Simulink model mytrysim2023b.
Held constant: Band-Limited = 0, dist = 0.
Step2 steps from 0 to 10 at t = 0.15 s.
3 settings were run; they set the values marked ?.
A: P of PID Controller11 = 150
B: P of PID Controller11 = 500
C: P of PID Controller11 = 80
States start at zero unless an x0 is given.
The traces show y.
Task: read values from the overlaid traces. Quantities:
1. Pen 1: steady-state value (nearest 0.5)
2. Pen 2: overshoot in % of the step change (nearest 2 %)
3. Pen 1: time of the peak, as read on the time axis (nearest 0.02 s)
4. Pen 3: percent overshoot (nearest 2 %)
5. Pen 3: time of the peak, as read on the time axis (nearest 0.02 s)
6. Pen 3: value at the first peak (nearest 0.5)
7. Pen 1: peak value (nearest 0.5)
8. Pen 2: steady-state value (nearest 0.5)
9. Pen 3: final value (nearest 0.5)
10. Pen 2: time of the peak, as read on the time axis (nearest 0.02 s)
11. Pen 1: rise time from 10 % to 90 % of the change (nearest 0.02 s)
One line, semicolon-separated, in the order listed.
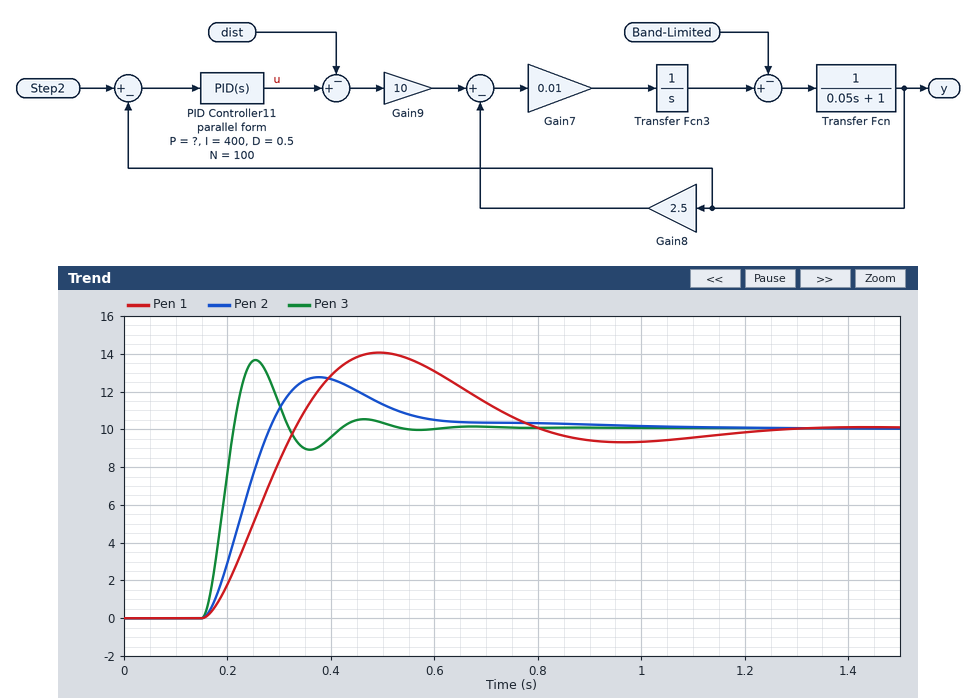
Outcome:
10.0; 28 %; 0.50 s; 36 %; 0.26 s; 13.5; 14.0; 10.0; 10.0; 0.38 s; 0.12 s
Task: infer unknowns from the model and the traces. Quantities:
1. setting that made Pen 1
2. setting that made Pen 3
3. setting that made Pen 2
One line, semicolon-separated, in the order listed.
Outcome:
C; B; A
